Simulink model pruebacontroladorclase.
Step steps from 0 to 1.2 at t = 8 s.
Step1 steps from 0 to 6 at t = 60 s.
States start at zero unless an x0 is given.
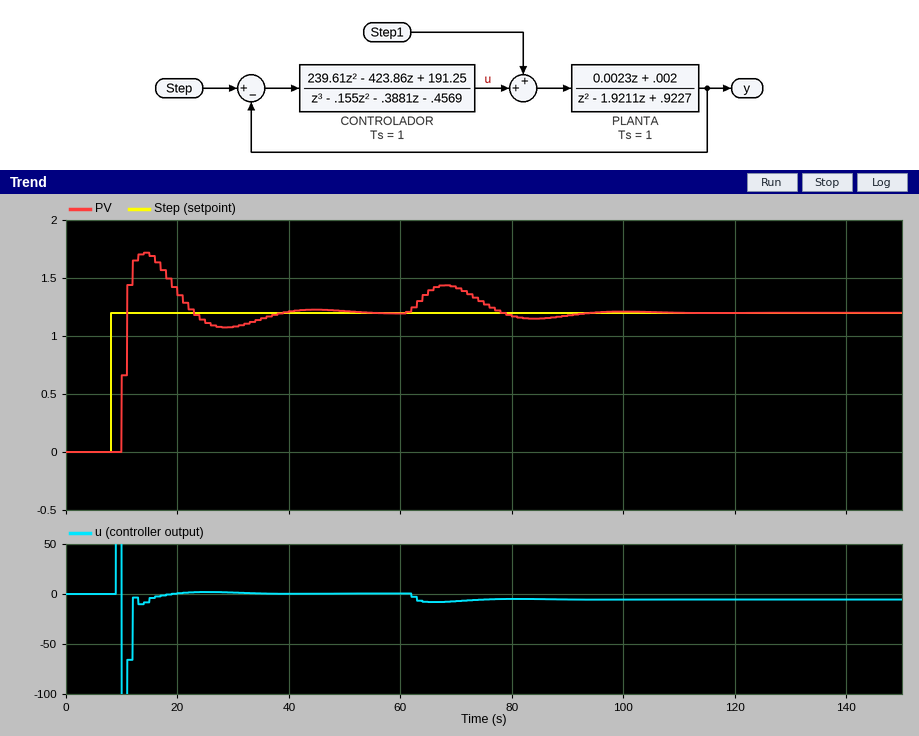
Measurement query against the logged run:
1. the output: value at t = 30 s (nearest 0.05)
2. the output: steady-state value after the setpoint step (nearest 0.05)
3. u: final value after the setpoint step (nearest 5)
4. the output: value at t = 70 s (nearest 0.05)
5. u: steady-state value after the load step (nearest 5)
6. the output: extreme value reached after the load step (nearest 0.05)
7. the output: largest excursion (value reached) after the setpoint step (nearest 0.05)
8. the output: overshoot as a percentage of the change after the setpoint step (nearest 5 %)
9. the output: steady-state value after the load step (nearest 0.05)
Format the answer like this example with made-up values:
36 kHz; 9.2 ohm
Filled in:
1.10; 1.20; 0; 1.40; -5; 1.45; 1.70; 45 %; 1.20
